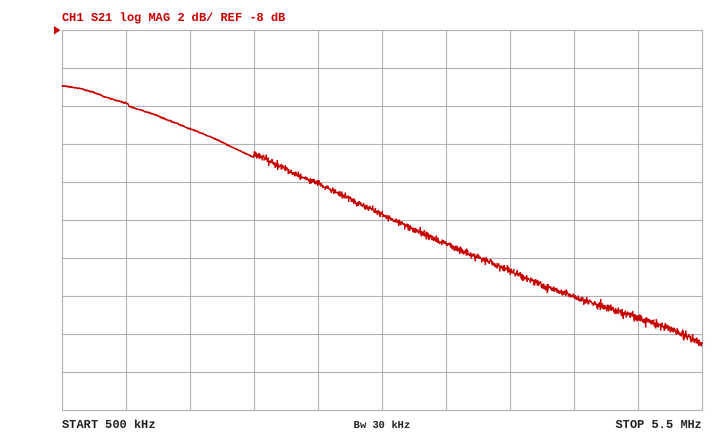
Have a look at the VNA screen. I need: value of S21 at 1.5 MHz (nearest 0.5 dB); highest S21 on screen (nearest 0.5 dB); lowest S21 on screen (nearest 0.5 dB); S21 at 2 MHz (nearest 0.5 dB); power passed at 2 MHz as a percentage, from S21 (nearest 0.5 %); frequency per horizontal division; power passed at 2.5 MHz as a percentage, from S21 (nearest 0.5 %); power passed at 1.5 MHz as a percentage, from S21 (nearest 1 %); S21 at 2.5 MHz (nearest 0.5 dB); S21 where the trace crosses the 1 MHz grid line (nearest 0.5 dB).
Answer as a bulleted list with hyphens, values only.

- -13.0 dB
- -11.0 dB
- -24.5 dB
- -14.5 dB
- 3.5 %
- 500 kHz
- 2.5 %
- 5 %
- -16.0 dB
- -12.0 dB
